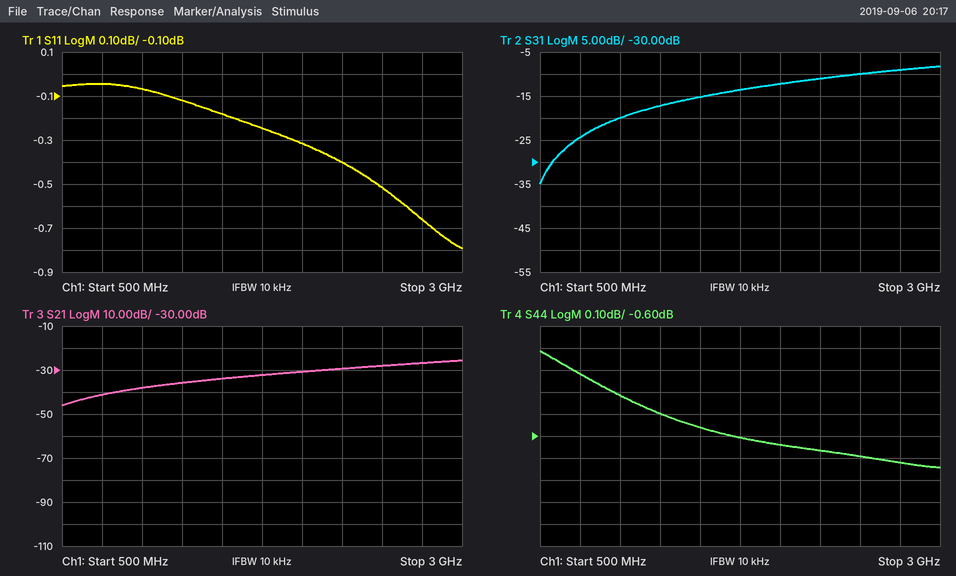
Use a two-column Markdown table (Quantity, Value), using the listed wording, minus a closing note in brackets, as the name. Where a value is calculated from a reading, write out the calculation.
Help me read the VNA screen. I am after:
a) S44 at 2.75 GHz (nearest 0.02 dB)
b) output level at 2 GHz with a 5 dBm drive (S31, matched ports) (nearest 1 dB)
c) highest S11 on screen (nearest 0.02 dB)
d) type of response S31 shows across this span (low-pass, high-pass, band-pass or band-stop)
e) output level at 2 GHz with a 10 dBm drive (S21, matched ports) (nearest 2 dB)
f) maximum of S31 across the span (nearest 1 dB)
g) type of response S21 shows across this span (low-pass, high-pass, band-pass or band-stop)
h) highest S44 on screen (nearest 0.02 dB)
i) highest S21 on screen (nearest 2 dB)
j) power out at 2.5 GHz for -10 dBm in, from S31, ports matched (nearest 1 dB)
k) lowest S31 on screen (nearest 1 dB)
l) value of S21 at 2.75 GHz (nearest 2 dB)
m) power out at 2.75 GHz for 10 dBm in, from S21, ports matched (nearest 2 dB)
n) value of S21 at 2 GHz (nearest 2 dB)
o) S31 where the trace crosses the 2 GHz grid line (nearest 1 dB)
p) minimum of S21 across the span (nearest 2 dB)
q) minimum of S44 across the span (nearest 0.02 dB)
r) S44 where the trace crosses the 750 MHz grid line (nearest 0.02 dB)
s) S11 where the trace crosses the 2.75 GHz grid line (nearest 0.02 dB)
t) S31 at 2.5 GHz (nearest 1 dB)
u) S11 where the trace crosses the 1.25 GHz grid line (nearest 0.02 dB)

| Quantity | Value |
|---|---|
| S44 at 2.75 GHz | -0.72 dB |
| output level at 2 GHz with a 5 dBm drive (S31, matched ports) | 5 dBm + (-12 dB) = -7 dBm |
| highest S11 on screen | -0.04 dB |
| type of response S31 shows across this span | high-pass |
| output level at 2 GHz with a 10 dBm drive (S21, matched ports) | 10 dBm + (-30 dB) = -20 dBm |
| maximum of S31 across the span | -8 dB |
| type of response S21 shows across this span | high-pass |
| highest S44 on screen | -0.22 dB |
| highest S21 on screen | -26 dB |
| power out at 2.5 GHz for -10 dBm in, from S31, ports matched | -10 dBm + (-10 dB) = -20 dBm |
| lowest S31 on screen | -35 dB |
| value of S21 at 2.75 GHz | -26 dB |
| power out at 2.75 GHz for 10 dBm in, from S21, ports matched | 10 dBm + (-26 dB) = -16 dBm |
| value of S21 at 2 GHz | -30 dB |
| S31 where the trace crosses the 2 GHz grid line | -12 dB |
| minimum of S21 across the span | -46 dB |
| minimum of S44 across the span | -0.74 dB |
| S44 where the trace crosses the 750 MHz grid line | -0.32 dB |
| S11 where the trace crosses the 2.75 GHz grid line | -0.66 dB |
| S31 at 2.5 GHz | -10 dB |
| S11 where the trace crosses the 1.25 GHz grid line | -0.12 dB |
